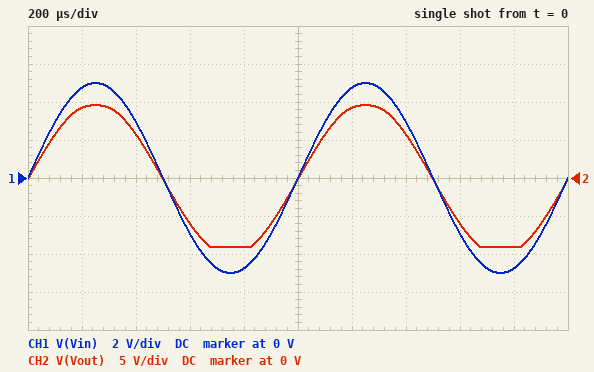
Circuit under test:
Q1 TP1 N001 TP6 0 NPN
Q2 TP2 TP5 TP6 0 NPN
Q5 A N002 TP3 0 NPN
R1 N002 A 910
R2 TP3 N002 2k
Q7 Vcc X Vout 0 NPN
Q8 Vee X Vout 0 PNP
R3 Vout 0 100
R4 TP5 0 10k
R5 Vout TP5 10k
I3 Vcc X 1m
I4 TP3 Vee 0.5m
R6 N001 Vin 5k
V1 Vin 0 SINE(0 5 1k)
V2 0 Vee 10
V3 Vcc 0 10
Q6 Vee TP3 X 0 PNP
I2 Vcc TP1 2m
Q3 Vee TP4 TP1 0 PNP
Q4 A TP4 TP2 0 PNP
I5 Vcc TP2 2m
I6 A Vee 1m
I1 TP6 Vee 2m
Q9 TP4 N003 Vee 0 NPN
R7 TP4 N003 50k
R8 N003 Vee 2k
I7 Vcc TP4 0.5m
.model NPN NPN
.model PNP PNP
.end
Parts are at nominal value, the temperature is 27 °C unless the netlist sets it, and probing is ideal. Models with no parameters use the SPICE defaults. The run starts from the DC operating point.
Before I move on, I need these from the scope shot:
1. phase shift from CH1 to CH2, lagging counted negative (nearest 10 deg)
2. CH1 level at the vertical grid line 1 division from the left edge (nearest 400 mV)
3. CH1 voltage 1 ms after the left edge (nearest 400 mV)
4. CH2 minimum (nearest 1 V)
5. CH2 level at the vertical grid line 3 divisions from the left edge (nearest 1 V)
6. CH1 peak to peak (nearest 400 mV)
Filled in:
0 deg
4.8 V
0 V
-9 V
-6 V
10.0 V
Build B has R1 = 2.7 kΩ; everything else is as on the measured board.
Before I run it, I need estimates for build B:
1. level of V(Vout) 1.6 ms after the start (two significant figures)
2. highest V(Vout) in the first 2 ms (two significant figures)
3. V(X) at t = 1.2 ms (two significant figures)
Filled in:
-6.0 V
9.0 V
9.9 V
